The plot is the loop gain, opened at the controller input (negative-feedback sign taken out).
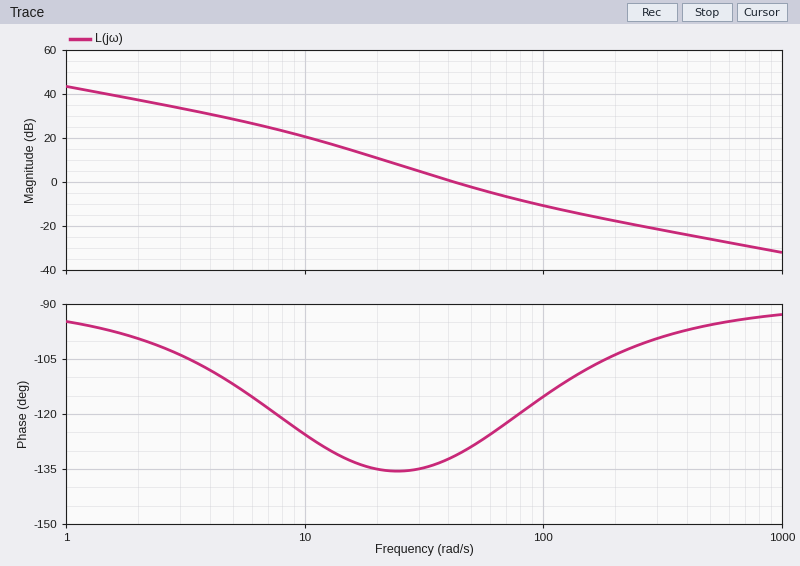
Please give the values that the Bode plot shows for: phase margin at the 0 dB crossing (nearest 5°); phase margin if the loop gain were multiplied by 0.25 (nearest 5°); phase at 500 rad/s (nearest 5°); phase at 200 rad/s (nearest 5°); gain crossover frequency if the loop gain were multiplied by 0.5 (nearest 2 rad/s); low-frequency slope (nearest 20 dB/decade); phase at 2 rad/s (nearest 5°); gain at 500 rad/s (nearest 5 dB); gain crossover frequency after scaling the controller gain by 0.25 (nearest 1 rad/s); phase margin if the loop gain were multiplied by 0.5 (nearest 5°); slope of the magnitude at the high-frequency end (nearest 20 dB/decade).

50°
45°
-95°
-105°
28 rad/s
-20 dB/decade
-100°
-25 dB
19 rad/s
45°
-20 dB/decade
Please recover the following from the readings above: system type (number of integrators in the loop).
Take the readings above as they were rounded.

1
